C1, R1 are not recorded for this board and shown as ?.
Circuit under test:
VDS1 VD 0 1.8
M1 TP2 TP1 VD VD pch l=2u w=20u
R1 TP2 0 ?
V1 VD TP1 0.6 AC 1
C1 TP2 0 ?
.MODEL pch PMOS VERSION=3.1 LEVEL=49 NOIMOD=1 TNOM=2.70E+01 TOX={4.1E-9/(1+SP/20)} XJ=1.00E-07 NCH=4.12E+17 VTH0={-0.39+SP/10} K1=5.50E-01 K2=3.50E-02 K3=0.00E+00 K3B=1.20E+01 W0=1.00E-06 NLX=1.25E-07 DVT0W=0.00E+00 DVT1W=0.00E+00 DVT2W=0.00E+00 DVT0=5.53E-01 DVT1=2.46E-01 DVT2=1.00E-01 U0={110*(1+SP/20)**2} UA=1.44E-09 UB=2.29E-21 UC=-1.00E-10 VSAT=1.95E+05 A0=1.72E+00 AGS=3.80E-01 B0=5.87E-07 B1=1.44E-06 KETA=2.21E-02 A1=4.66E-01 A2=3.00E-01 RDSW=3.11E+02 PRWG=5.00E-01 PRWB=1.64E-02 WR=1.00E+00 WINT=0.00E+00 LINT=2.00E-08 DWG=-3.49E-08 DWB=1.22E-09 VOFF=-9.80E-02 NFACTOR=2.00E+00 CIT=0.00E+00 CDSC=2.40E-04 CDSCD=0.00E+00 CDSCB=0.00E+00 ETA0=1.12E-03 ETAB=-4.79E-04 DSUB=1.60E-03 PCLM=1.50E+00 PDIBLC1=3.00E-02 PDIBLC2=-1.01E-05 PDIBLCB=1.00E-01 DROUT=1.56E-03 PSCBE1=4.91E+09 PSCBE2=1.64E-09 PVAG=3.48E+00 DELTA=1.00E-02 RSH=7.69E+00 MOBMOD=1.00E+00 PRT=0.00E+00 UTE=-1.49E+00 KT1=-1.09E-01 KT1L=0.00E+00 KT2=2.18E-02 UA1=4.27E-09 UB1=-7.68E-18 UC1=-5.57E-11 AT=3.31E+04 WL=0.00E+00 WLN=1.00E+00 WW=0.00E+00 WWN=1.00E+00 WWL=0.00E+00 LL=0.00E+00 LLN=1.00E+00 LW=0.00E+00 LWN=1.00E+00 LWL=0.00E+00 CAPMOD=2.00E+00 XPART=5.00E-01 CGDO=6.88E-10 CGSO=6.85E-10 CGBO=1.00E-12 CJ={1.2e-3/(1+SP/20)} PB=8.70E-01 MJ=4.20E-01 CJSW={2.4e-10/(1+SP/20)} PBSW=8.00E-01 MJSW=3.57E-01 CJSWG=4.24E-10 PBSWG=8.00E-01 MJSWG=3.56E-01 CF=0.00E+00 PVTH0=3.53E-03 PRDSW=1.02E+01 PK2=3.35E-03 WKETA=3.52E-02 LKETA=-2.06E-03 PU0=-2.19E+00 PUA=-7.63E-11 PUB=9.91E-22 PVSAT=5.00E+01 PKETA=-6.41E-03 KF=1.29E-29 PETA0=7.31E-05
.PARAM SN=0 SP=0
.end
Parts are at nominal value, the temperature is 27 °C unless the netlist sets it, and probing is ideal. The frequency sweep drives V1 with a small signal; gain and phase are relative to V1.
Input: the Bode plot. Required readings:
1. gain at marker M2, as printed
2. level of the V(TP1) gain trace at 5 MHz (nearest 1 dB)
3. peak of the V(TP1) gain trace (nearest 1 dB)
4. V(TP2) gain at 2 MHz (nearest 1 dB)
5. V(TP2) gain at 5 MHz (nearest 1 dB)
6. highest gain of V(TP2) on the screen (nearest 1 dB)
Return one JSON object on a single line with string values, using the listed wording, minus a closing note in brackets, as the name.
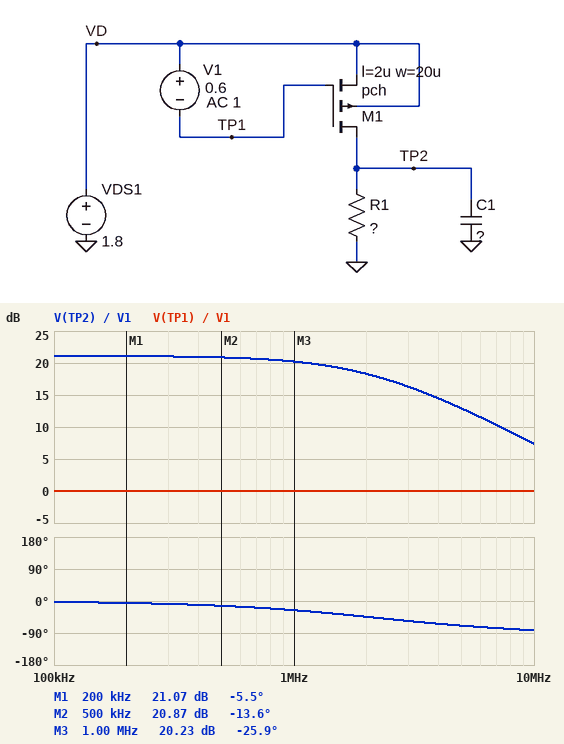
{"gain at marker M2, as printed": "20.87 dB", "level of the V(TP1) gain trace at 5 MHz": "0 dB", "peak of the V(TP1) gain trace": "0 dB", "V(TP2) gain at 2 MHz": "18 dB", "V(TP2) gain at 5 MHz": "13 dB", "highest gain of V(TP2) on the screen": "21 dB"}
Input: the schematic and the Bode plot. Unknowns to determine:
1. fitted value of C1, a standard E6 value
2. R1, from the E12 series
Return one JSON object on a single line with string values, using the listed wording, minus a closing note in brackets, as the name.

{"fitted value of C1, a standard E6 value": "680 fF", "R1, from the E12 series": "120 kΩ"}
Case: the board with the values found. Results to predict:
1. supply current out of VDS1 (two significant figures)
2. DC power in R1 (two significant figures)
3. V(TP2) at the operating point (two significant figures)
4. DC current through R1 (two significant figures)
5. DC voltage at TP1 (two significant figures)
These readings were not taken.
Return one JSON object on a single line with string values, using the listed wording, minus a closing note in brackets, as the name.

{"supply current out of VDS1": "11 µA", "DC power in R1": "14 µW", "V(TP2) at the operating point": "1.3 V", "DC current through R1": "11 µA", "DC voltage at TP1": "1.2 V"}
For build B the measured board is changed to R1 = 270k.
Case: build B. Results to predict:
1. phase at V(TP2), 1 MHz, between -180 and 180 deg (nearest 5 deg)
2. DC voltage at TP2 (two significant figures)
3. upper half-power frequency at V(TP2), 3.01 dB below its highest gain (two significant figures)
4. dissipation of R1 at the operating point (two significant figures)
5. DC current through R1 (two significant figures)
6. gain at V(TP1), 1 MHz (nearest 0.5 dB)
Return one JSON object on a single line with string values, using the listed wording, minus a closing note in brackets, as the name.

{"phase at V(TP2), 1 MHz, between -180 and 180 deg": "-5 deg", "DC voltage at TP2": "1.7 V", "upper half-power frequency at V(TP2), 3.01 dB below its highest gain": "18 MHz", "dissipation of R1 at the operating point": "11 µW", "DC current through R1": "6.4 µA", "gain at V(TP1), 1 MHz": "0 dB"}
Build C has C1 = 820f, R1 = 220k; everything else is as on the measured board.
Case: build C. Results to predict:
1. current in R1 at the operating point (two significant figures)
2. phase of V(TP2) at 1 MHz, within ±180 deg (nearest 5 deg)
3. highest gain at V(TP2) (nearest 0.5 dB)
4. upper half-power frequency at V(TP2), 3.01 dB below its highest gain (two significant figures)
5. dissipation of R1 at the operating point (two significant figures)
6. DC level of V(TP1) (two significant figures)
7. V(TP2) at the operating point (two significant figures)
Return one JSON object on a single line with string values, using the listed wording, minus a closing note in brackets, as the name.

{"current in R1 at the operating point": "7.8 µA", "phase of V(TP2) at 1 MHz, within ±180 deg": "-5 deg", "highest gain at V(TP2)": "-0.5 dB", "upper half-power frequency at V(TP2), 3.01 dB below its highest gain": "11 MHz", "dissipation of R1 at the operating point": "13 µW", "DC level of V(TP1)": "1.2 V", "V(TP2) at the operating point": "1.7 V"}
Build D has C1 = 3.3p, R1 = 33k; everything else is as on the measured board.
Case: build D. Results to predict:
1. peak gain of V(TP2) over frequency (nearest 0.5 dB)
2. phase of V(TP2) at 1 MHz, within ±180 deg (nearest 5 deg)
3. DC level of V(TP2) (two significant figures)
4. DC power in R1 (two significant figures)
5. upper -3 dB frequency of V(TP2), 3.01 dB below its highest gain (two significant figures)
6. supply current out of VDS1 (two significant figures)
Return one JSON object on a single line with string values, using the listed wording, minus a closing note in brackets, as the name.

{"peak gain of V(TP2) over frequency": "11.0 dB", "phase of V(TP2) at 1 MHz, within ±180 deg": "-35 deg", "DC level of V(TP2)": "390 mV", "DC power in R1": "4.6 µW", "upper -3 dB frequency of V(TP2), 3.01 dB below its highest gain": "1.5 MHz", "supply current out of VDS1": "12 µA"}
